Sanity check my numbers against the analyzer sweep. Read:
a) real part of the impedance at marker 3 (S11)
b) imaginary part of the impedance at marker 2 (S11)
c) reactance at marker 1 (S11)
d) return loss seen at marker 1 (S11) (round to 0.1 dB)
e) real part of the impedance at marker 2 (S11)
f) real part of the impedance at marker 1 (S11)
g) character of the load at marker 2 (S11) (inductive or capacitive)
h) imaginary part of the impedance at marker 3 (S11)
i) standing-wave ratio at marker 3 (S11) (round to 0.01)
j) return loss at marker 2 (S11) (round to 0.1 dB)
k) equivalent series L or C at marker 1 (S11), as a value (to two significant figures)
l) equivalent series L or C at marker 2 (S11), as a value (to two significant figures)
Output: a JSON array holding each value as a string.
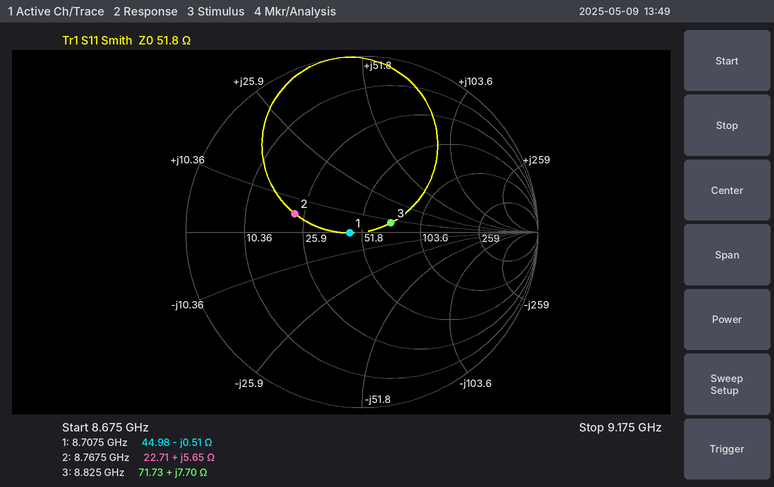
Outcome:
["71.73 Ω", "+5.65 Ω", "-0.51 Ω", "23.0 dB", "22.71 Ω", "44.98 Ω", "inductive", "+7.70 Ω", "1.42", "8.0 dB", "36 pF", "100 pH"]
